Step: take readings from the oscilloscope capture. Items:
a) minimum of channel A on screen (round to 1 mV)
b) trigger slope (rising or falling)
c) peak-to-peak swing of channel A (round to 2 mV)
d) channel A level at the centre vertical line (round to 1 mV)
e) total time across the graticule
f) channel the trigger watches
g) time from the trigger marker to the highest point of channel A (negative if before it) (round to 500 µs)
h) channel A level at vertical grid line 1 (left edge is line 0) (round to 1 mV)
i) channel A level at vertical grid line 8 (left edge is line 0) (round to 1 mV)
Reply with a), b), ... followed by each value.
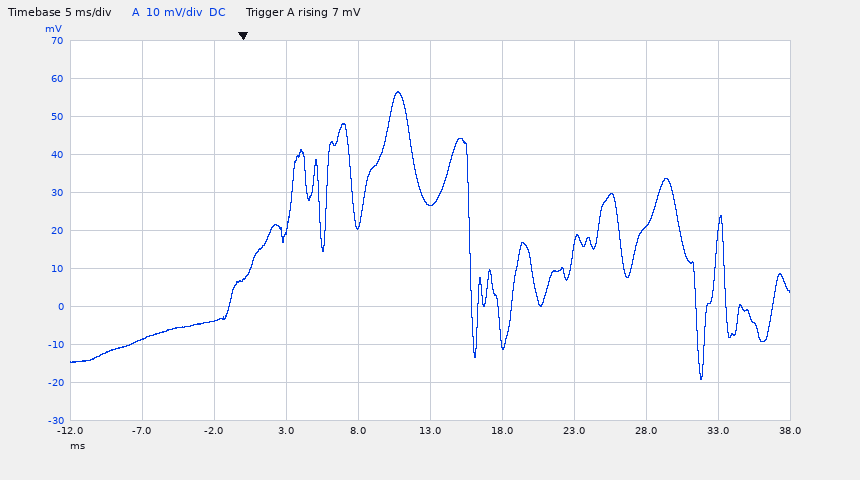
a) -19 mV
b) rising
c) 76 mV
d) 27 mV
e) 50 ms
f) channel A
g) +11.0 ms
h) -9 mV
i) 21 mV
